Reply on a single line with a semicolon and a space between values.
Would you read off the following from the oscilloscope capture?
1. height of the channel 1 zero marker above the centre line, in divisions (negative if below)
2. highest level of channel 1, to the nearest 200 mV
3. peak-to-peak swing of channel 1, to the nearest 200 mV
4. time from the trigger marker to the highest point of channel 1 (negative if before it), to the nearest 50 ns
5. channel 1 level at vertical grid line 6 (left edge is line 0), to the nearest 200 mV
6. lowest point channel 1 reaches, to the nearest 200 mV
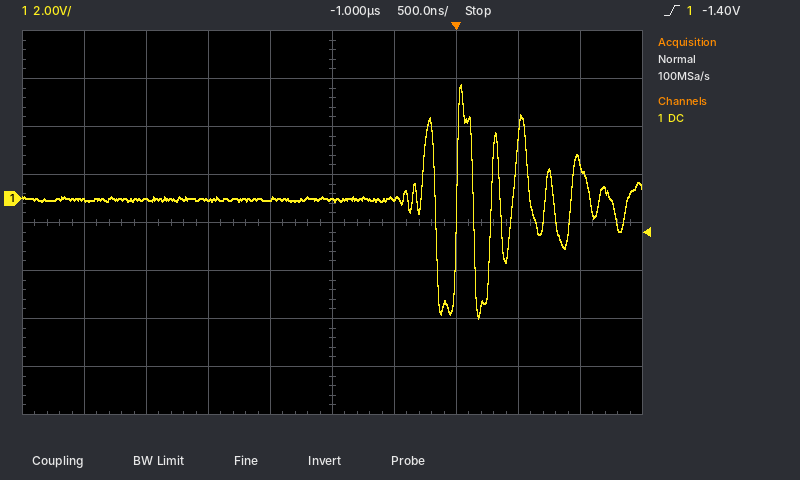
+0.5 div; 4.8 V; 9.8 V; +50 ns; 0.0 V; -5.0 V
